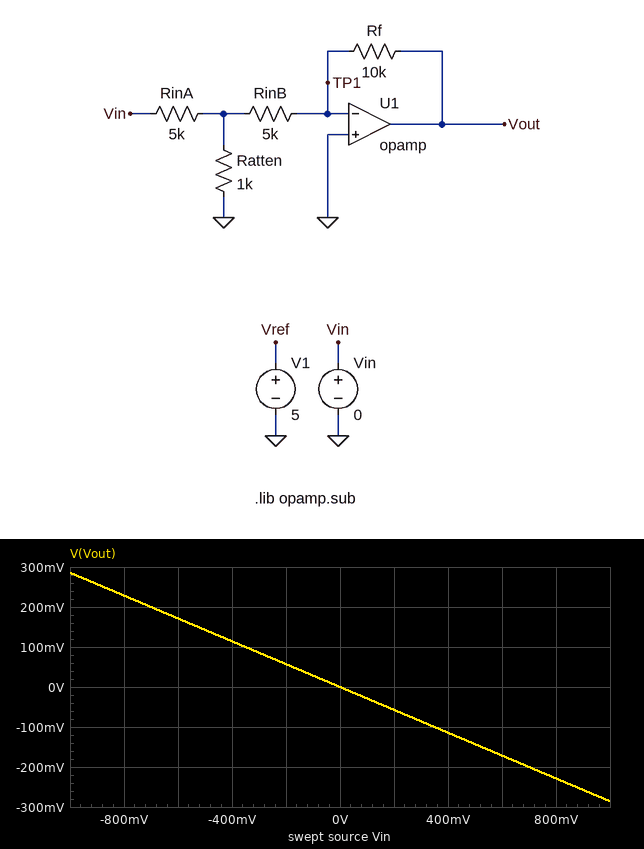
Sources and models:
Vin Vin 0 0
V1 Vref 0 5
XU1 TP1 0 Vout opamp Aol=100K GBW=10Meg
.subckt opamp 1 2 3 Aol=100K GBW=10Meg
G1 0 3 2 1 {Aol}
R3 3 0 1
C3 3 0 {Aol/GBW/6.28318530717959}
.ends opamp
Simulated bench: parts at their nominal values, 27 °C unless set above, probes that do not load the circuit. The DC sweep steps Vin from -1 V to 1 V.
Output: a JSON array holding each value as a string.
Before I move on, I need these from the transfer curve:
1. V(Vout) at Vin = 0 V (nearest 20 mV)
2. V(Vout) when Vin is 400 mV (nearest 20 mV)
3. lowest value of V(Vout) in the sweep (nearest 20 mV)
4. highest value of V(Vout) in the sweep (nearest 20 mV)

["0 V", "-120 mV", "-280 mV", "280 mV"]
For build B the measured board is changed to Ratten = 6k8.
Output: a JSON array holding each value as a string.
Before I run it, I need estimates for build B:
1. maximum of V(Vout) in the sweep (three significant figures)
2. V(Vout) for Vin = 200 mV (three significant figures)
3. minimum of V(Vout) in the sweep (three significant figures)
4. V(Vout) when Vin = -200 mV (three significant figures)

["731 mV", "-146 mV", "-731 mV", "146 mV"]
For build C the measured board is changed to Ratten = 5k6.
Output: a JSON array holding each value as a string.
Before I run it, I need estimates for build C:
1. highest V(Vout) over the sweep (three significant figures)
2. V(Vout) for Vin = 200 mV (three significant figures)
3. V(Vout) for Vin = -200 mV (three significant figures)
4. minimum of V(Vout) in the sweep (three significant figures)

["691 mV", "-138 mV", "138 mV", "-691 mV"]
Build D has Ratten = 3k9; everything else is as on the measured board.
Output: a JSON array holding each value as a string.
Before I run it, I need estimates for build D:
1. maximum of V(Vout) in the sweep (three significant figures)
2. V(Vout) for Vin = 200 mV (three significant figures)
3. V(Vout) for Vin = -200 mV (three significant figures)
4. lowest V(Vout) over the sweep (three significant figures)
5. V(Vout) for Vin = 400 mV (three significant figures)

["609 mV", "-122 mV", "122 mV", "-609 mV", "-244 mV"]
